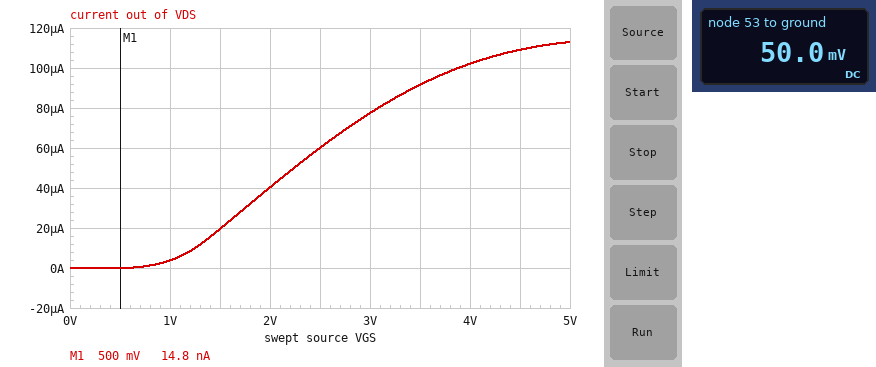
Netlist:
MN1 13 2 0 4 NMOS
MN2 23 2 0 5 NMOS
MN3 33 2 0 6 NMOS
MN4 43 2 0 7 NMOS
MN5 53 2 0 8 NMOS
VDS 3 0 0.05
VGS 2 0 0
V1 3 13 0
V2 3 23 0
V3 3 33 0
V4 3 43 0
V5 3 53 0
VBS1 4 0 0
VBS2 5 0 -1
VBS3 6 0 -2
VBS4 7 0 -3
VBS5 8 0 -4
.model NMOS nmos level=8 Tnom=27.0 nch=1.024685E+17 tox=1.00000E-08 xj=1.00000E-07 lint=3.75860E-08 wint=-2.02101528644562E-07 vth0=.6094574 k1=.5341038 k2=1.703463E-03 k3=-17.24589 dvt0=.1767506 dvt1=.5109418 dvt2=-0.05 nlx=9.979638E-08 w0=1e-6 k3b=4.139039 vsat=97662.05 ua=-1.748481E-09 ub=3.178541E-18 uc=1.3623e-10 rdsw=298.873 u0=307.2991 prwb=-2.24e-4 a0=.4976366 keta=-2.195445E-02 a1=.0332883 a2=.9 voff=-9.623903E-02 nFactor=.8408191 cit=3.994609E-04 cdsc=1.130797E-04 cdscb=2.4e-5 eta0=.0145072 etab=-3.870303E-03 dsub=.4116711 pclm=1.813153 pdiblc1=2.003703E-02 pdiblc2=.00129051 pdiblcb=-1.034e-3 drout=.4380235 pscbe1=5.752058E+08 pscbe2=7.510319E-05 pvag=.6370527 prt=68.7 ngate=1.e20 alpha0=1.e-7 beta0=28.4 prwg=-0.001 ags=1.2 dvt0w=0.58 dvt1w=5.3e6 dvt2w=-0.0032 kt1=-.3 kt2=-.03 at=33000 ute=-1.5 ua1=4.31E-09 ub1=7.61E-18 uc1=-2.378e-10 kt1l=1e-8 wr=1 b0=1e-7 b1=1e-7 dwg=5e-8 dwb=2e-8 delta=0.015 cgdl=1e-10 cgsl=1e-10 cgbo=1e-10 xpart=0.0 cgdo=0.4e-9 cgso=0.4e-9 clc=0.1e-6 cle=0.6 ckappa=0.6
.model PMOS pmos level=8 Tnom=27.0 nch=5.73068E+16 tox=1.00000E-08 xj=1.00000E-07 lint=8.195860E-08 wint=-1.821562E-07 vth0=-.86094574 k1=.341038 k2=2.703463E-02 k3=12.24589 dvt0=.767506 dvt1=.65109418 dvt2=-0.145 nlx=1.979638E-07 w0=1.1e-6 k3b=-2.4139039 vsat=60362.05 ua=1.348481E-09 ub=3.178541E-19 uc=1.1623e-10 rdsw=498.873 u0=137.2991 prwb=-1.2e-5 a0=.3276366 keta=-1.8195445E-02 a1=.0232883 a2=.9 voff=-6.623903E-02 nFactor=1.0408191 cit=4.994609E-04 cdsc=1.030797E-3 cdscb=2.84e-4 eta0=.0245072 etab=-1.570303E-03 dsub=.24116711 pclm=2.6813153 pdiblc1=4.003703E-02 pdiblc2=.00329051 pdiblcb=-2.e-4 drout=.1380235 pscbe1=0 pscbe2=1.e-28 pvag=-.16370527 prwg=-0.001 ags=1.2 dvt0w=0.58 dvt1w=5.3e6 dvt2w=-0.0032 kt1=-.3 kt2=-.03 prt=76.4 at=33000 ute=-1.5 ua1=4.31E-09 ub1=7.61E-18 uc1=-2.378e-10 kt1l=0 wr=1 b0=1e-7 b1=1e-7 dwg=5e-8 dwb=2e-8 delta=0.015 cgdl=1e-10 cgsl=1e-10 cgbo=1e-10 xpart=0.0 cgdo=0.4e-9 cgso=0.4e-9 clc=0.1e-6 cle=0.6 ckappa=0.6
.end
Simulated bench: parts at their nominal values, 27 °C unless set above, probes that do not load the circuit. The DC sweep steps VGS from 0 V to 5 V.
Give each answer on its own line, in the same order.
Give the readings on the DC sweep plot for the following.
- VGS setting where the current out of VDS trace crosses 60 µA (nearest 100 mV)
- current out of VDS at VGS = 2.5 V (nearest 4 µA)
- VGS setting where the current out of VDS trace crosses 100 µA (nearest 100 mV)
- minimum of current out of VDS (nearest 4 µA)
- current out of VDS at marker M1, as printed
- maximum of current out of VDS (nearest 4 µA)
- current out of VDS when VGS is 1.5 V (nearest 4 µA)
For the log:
2.5 V
60 µA
3.9 V
0 A
14.8 nA
112 µA
20 µA
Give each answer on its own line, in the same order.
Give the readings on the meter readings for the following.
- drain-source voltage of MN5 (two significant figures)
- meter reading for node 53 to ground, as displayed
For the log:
50 mV
50.0 mV
